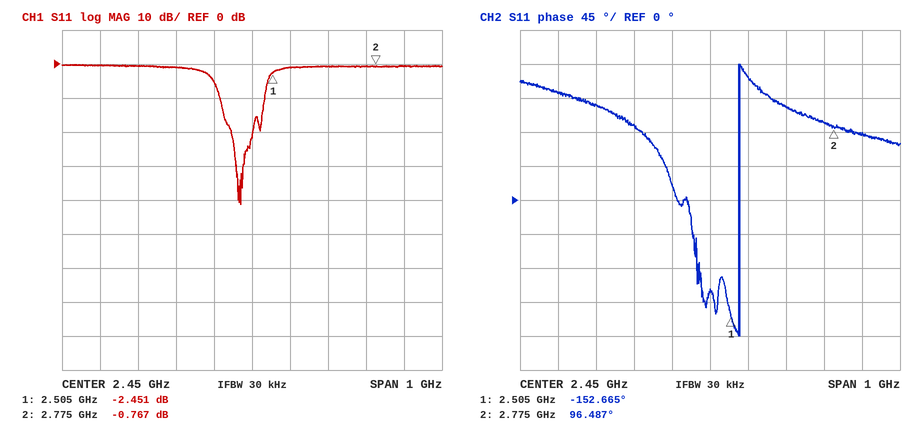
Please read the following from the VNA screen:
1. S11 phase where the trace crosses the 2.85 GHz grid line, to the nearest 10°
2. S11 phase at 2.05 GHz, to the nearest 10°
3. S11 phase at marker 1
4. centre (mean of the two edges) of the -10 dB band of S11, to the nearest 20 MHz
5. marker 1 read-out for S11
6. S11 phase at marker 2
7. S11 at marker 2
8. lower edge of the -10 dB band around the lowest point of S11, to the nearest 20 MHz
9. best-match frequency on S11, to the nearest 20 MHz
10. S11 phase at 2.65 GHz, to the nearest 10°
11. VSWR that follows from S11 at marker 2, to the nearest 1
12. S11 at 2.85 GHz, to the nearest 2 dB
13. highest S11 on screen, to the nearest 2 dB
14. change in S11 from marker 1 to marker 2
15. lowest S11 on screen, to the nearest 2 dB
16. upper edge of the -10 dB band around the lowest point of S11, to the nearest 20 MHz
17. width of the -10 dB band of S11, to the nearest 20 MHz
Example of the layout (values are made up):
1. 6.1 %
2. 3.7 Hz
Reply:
1. 90°
2. 140°
3. -152.665°
4. 2.42 GHz
5. -2.451 dB
6. 96.487°
7. -0.767 dB
8. 2.36 GHz
9. 2.42 GHz
10. 120°
11. 23
12. 0 dB
13. 0 dB
14. 1.684 dB
15. -42 dB
16. 2.48 GHz
17. 120 MHz
